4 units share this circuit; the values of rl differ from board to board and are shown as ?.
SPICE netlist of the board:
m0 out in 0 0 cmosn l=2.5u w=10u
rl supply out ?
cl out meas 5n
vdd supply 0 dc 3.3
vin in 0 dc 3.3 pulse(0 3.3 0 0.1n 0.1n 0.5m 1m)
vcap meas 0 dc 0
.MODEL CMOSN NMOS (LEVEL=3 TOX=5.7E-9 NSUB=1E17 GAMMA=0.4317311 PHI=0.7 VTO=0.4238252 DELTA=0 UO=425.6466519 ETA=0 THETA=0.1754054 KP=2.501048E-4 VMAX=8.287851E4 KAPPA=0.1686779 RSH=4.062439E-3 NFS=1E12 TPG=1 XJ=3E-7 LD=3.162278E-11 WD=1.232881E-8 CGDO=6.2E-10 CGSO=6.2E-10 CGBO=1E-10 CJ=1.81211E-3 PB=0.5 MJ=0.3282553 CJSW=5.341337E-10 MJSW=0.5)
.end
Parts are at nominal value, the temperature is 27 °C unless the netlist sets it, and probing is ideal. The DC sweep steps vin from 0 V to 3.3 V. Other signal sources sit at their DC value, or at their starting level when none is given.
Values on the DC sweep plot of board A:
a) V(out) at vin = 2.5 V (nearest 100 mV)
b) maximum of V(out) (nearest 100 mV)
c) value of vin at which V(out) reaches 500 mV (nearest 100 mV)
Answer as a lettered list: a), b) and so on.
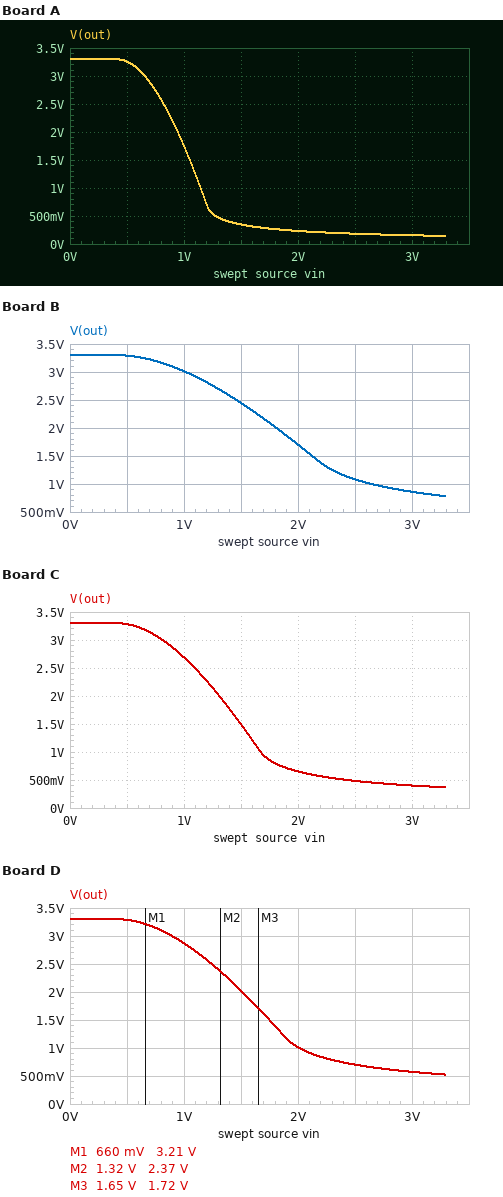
a) 200 mV
b) 3.3 V
c) 1.3 V
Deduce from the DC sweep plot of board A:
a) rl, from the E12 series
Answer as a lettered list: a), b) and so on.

a) 12 kΩ
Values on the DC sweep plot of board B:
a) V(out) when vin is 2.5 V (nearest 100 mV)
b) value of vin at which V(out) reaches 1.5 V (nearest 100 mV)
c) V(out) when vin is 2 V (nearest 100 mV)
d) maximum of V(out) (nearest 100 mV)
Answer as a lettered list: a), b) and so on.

a) 1.1 V
b) 2.1 V
c) 1.7 V
d) 3.3 V
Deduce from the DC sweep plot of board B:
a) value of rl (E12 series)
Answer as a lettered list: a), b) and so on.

a) 2.2 kΩ
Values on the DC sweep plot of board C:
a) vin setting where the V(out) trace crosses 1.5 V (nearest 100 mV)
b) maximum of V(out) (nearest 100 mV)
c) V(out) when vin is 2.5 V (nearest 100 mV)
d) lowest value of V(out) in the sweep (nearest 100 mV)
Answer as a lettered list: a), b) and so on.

a) 1.5 V
b) 3.3 V
c) 500 mV
d) 400 mV
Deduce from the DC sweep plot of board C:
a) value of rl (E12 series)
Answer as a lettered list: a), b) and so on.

a) 4.7 kΩ
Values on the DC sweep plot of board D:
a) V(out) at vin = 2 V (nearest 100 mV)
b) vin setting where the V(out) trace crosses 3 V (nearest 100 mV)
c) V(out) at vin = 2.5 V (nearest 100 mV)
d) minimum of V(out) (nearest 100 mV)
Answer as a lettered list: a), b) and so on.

a) 1.0 V
b) 900 mV
c) 700 mV
d) 500 mV
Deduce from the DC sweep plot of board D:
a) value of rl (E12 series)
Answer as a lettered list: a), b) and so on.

a) 3.3 kΩ
